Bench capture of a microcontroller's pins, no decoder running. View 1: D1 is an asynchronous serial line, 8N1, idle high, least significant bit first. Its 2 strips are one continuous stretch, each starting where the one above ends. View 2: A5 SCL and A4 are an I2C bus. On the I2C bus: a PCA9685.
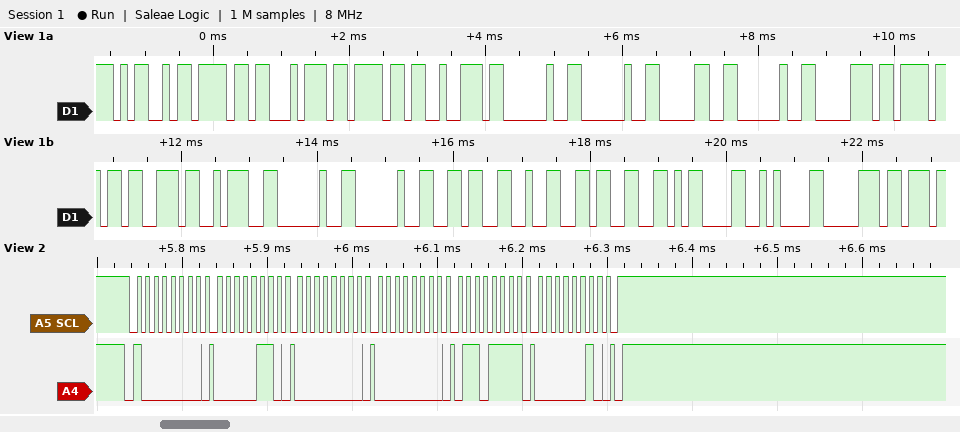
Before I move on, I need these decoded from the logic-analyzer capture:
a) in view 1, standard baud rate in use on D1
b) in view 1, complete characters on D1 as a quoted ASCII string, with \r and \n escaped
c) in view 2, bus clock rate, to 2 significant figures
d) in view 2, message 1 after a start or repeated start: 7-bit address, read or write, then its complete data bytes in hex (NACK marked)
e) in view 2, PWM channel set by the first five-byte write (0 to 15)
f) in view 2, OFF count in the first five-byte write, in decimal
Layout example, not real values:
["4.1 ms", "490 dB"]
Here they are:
["9600 baud", "\"Motor  0 pos:  623\\r\\np\"", "100 kHz", "0x40 write: 06 00 00 6F 02", "0", "623"]
